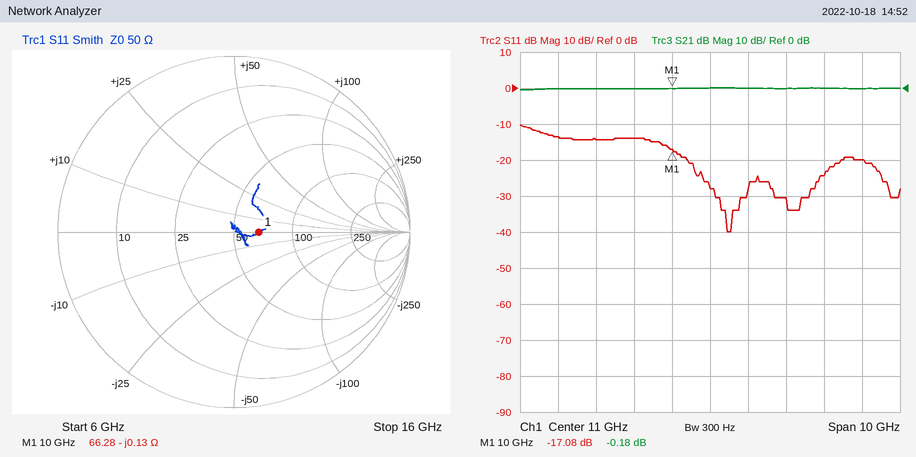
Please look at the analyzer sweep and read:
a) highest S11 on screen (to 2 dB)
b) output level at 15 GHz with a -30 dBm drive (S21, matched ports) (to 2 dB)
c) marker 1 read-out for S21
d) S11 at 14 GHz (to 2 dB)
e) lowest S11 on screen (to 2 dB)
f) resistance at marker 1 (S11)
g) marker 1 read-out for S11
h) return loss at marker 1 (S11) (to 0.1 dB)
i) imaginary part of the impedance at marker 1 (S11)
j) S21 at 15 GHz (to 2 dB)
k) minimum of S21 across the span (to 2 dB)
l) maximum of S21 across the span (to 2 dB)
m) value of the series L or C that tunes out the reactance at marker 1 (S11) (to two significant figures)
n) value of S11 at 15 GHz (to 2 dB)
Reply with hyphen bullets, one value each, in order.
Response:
- -10 dB
- -30 dBm
- -0.18 dB
- -24 dB
- -40 dB
- 66.28 Ω
- -17.08 dB
- 17.1 dB
- -0.13 Ω
- 0 dB
- 0 dB
- 0 dB
- 2.1 pH
- -20 dB
